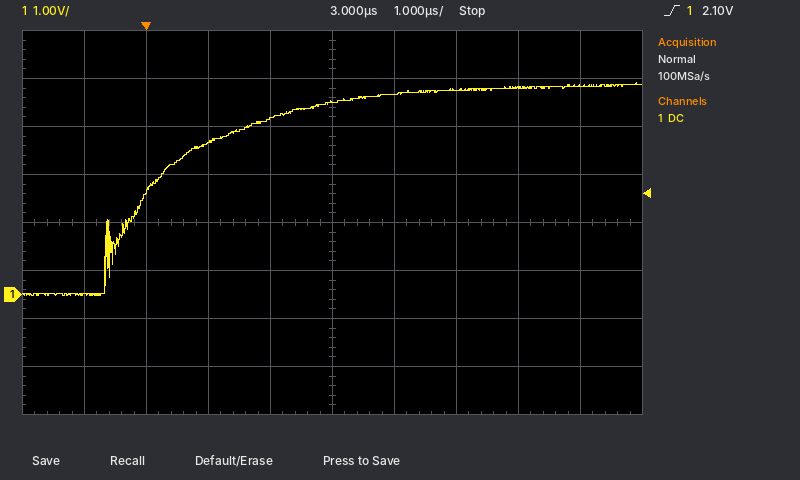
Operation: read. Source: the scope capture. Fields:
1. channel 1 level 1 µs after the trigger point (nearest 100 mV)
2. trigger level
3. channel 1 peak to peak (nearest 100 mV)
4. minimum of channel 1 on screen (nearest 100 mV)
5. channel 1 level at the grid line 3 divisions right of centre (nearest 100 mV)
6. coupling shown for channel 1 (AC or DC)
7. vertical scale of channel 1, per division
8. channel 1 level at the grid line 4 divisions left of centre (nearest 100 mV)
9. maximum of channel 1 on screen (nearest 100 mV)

3.2 V
2.10 V
4.4 V
0.0 V
4.3 V
DC
1 V
0.0 V
4.4 V
